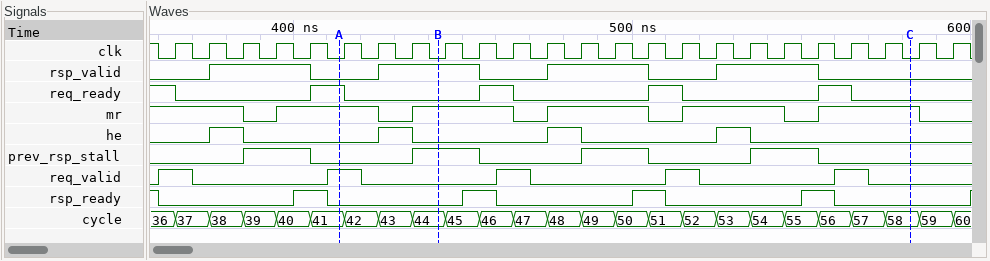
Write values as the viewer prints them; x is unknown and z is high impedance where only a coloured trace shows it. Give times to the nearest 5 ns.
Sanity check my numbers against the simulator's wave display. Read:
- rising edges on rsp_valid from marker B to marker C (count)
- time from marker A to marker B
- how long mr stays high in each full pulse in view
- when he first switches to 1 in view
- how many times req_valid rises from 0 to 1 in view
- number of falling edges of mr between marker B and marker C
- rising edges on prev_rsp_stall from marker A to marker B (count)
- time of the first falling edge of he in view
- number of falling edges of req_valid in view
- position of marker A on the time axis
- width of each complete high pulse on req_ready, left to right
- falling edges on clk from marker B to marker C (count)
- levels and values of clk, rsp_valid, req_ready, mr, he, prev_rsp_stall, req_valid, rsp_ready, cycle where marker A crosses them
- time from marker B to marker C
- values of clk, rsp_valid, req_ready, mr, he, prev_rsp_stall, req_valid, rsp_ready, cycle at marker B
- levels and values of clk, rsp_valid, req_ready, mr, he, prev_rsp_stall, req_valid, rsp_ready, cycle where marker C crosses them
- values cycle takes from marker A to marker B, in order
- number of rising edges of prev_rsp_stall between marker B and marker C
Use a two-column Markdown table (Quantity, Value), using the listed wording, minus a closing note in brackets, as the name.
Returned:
| Quantity | Value |
|---|---|
| rising edges on rsp_valid from marker B to marker C | 2 |
| time from marker A to marker B | 30 ns |
| how long mr stays high in each full pulse in view | 30 ns, 30 ns, 30 ns, 30 ns, 30 ns |
| when he first switches to 1 in view | 375 ns |
| how many times req_valid rises from 0 to 1 in view | 5 |
| number of falling edges of mr between marker B and marker C | 3 |
| rising edges on prev_rsp_stall from marker A to marker B | 1 |
| time of the first falling edge of he in view | 385 ns |
| number of falling edges of req_valid in view | 5 |
| position of marker A on the time axis | 415 ns |
| width of each complete high pulse on req_ready, left to right | 10 ns, 10 ns, 10 ns, 10 ns |
| falling edges on clk from marker B to marker C | 14 |
| levels and values of clk, rsp_valid, req_ready, mr, he, prev_rsp_stall, req_valid, rsp_ready, cycle where marker A crosses them | clk=0, rsp_valid=0, req_ready=1, mr=1, he=0, prev_rsp_stall=0, req_valid=1, rsp_ready=0, cycle=41 |
| time from marker B to marker C | 140 ns |
| values of clk, rsp_valid, req_ready, mr, he, prev_rsp_stall, req_valid, rsp_ready, cycle at marker B | clk=0, rsp_valid=1, req_ready=0, mr=1, he=0, prev_rsp_stall=1, req_valid=0, rsp_ready=0, cycle=44 |
| levels and values of clk, rsp_valid, req_ready, mr, he, prev_rsp_stall, req_valid, rsp_ready, cycle where marker C crosses them | clk=0, rsp_valid=0, req_ready=0, mr=1, he=0, prev_rsp_stall=0, req_valid=0, rsp_ready=0, cycle=58 |
| values cycle takes from marker A to marker B, in order | 41, 42, 43, 44 |
| number of rising edges of prev_rsp_stall between marker B and marker C | 2 |
